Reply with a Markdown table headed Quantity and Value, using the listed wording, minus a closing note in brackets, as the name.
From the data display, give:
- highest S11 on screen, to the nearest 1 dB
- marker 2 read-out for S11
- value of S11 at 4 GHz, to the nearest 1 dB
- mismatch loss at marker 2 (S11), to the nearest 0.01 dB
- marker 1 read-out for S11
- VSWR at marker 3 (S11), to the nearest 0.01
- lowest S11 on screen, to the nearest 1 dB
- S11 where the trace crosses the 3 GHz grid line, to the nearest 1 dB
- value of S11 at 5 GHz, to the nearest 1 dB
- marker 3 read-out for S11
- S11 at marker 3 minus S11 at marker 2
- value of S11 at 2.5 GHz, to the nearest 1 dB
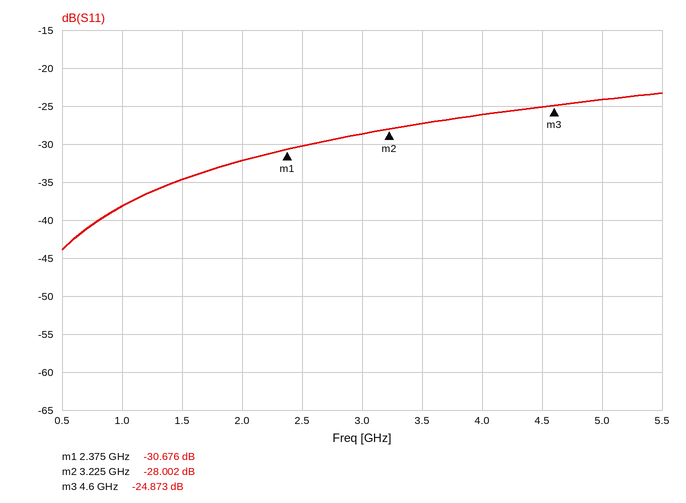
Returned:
| Quantity | Value |
|---|---|
| highest S11 on screen, to the nearest 1 dB | -23 dB |
| marker 2 read-out for S11 | -28.002 dB |
| value of S11 at 4 GHz, to the nearest 1 dB | -26 dB |
| mismatch loss at marker 2 (S11), to the nearest 0.01 dB | 0.01 dB |
| marker 1 read-out for S11 | -30.676 dB |
| VSWR at marker 3 (S11), to the nearest 0.01 | 1.12 |
| lowest S11 on screen, to the nearest 1 dB | -44 dB |
| S11 where the trace crosses the 3 GHz grid line, to the nearest 1 dB | -29 dB |
| value of S11 at 5 GHz, to the nearest 1 dB | -24 dB |
| marker 3 read-out for S11 | -24.873 dB |
| S11 at marker 3 minus S11 at marker 2 | 3.129 dB |
| value of S11 at 2.5 GHz, to the nearest 1 dB | -30 dB |
